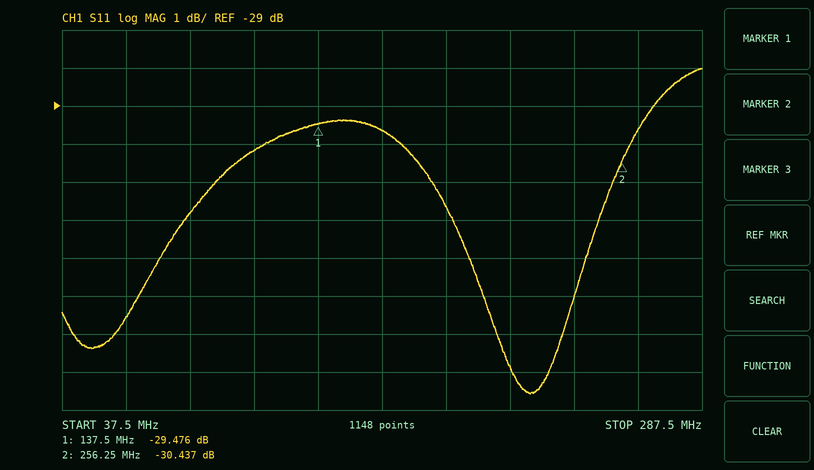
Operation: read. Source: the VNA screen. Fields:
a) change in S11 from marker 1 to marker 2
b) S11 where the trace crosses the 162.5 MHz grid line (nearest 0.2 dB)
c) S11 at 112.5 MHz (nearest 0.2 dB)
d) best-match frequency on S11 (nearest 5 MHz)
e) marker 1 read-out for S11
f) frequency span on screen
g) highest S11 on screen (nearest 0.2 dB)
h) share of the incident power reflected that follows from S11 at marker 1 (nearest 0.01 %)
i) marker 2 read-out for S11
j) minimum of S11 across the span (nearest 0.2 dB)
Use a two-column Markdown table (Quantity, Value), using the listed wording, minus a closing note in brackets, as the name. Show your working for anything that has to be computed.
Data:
| Quantity | Value |
|---|---|
| change in S11 from marker 1 to marker 2 | -30.437 − (-29.476) = -0.961 dB |
| S11 where the trace crosses the 162.5 MHz grid line | -29.6 dB |
| S11 at 112.5 MHz | -30.2 dB |
| best-match frequency on S11 | 220 MHz |
| marker 1 read-out for S11 | -29.476 dB |
| frequency span on screen | 250 MHz |
| highest S11 on screen | -28.0 dB |
| share of the incident power reflected that follows from S11 at marker 1 | 10^(-29.476/10) ≈ 0.11 % |
| marker 2 read-out for S11 | -30.437 dB |
| minimum of S11 across the span | -36.6 dB |
